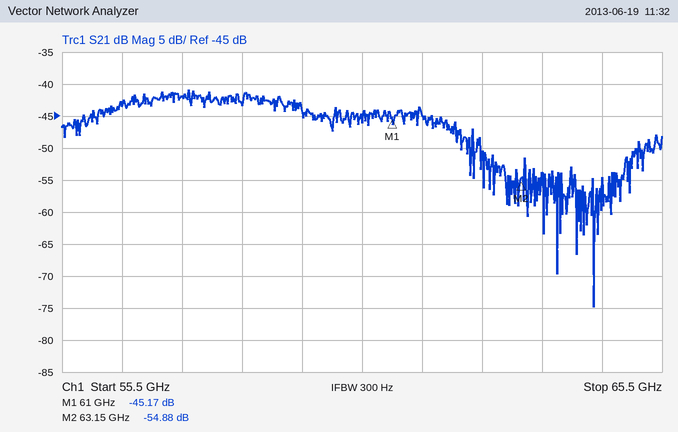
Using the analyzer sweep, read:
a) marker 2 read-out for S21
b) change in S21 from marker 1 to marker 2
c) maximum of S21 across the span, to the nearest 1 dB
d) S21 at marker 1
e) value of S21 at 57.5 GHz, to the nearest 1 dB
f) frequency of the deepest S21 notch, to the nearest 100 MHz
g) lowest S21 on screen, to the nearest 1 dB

-54.88 dB
-9.71 dB
-41 dB
-45.17 dB
-42 dB
64.4 GHz
-75 dB
